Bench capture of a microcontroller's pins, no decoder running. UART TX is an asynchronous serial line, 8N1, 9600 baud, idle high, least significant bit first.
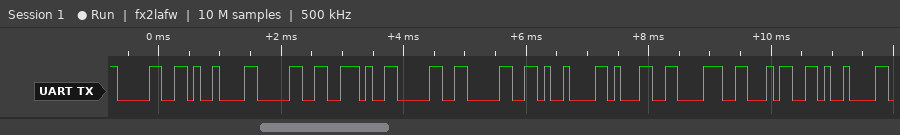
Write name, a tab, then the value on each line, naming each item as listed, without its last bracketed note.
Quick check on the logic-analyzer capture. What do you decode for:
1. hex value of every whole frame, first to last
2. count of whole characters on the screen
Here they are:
hex value of every whole frame, first to last	0x30 0x09 0x30 0x2E 0x30 0x30 0x09 0x31 0x38 0x34 0x09
count of whole characters on the screen	11
